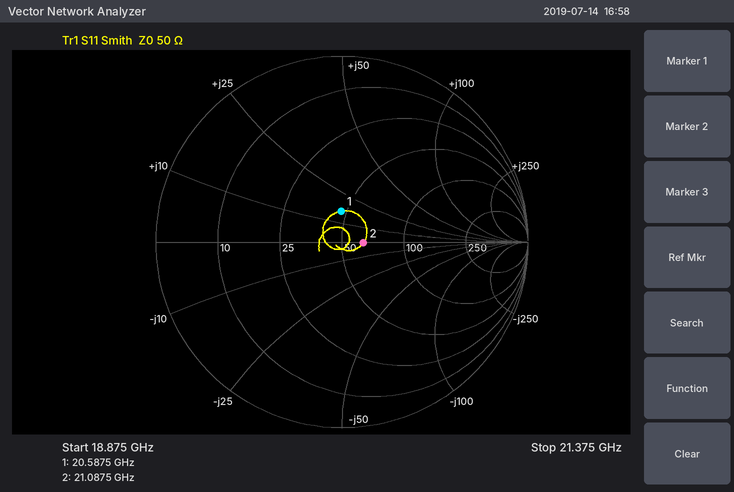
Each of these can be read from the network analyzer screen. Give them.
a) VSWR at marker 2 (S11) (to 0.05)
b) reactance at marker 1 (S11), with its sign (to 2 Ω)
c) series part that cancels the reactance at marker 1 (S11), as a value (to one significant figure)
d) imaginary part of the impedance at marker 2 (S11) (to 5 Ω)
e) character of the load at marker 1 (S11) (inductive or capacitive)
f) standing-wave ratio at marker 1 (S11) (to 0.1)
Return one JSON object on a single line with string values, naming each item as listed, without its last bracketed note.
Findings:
{"VSWR at marker 2 (S11)": "1.25", "reactance at marker 1 (S11), with its sign": "+16 Ω", "series part that cancels the reactance at marker 1 (S11), as a value": "500 fF", "imaginary part of the impedance at marker 2 (S11)": "0 Ω", "character of the load at marker 1 (S11)": "inductive", "standing-wave ratio at marker 1 (S11)": "1.4"}
